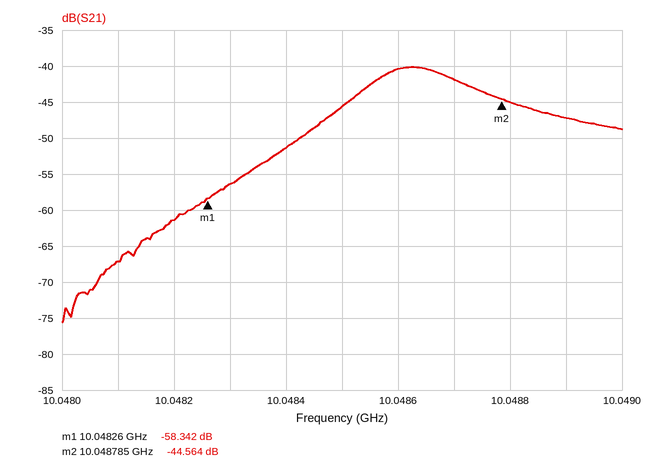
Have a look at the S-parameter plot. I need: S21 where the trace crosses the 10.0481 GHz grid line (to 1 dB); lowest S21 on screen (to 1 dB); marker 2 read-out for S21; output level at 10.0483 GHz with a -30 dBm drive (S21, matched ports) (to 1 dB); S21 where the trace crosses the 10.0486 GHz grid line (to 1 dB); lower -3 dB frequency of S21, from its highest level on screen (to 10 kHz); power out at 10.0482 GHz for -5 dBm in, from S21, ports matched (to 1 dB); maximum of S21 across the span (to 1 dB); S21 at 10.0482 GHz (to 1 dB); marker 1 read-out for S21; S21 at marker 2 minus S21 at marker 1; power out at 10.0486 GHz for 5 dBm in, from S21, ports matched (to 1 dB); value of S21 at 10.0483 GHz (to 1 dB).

-67 dB
-76 dB
-44.564 dB
-86 dBm
-40 dB
10.04854 GHz
-66 dBm
-40 dB
-61 dB
-58.342 dB
13.778 dB
-35 dBm
-56 dB
